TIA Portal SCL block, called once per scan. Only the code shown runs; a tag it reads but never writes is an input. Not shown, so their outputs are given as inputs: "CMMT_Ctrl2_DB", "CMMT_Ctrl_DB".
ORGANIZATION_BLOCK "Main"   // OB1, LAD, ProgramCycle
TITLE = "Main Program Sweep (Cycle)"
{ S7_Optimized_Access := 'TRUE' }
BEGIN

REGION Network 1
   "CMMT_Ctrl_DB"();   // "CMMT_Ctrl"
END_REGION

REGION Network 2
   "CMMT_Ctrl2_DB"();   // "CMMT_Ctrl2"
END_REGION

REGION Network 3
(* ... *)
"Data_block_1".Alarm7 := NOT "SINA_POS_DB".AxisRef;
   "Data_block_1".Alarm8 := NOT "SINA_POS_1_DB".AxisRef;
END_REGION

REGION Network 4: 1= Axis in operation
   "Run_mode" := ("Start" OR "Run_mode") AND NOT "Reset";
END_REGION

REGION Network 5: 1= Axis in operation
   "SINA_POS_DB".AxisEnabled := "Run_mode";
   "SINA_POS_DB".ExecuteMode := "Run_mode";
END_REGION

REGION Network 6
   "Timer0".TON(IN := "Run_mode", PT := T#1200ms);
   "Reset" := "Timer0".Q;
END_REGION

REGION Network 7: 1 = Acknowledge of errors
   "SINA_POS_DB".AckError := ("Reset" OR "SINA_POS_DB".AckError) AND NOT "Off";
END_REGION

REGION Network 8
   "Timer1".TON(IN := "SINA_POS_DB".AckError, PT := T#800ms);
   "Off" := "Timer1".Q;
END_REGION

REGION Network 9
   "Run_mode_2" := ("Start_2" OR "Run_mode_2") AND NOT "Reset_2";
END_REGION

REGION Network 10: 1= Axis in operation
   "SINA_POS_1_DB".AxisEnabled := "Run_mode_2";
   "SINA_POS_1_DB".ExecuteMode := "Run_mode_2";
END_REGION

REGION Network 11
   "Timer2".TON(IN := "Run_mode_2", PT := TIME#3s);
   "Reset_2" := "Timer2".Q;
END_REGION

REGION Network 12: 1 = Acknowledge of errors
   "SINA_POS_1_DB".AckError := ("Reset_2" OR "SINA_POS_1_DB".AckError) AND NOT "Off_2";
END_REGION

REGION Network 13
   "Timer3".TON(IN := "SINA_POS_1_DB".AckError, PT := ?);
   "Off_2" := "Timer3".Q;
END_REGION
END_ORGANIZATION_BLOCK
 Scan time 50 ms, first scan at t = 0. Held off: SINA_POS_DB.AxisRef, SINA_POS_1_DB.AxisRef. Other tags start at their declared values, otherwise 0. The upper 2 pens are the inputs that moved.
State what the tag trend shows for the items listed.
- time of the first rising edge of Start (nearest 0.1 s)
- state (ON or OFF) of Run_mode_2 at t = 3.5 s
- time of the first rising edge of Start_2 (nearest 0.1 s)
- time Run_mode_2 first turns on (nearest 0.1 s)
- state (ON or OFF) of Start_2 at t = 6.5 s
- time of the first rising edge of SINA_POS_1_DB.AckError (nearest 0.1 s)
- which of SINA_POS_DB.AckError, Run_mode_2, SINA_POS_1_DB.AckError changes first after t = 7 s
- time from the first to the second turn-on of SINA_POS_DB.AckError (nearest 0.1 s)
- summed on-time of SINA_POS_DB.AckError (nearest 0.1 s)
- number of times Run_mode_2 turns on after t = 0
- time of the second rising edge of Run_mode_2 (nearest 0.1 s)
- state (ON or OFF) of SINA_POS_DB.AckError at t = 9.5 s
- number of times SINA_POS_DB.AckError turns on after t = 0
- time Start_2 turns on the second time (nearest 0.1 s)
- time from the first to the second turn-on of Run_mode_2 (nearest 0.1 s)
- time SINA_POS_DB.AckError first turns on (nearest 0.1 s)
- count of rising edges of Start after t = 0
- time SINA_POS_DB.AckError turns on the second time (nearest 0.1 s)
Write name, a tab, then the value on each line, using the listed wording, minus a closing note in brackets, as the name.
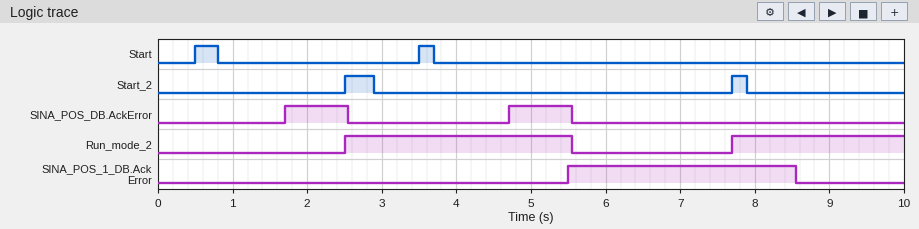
time of the first rising edge of Start	0.5 s
state (ON or OFF) of Run_mode_2 at t = 3.5 s	ON
time of the first rising edge of Start_2	2.5 s
time Run_mode_2 first turns on	2.5 s
state (ON or OFF) of Start_2 at t = 6.5 s	OFF
time of the first rising edge of SINA_POS_1_DB.AckError	5.5 s
which of SINA_POS_DB.AckError, Run_mode_2, SINA_POS_1_DB.AckError changes first after t = 7 s	Run_mode_2
time from the first to the second turn-on of SINA_POS_DB.AckError	3.0 s
summed on-time of SINA_POS_DB.AckError	1.7 s
number of times Run_mode_2 turns on after t = 0	2
time of the second rising edge of Run_mode_2	7.7 s
state (ON or OFF) of SINA_POS_DB.AckError at t = 9.5 s	OFF
number of times SINA_POS_DB.AckError turns on after t = 0	2
time Start_2 turns on the second time	7.7 s
time from the first to the second turn-on of Run_mode_2	5.2 s
time SINA_POS_DB.AckError first turns on	1.7 s
count of rising edges of Start after t = 0	2
time SINA_POS_DB.AckError turns on the second time	4.7 s
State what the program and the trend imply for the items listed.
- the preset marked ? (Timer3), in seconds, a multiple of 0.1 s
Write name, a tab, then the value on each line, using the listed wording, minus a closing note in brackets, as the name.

the preset marked ? (Timer3), in seconds, a multiple of 0.1 s	3.0 s
